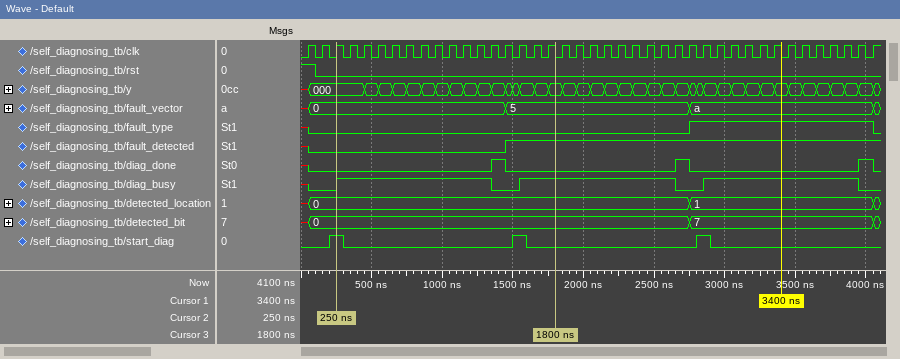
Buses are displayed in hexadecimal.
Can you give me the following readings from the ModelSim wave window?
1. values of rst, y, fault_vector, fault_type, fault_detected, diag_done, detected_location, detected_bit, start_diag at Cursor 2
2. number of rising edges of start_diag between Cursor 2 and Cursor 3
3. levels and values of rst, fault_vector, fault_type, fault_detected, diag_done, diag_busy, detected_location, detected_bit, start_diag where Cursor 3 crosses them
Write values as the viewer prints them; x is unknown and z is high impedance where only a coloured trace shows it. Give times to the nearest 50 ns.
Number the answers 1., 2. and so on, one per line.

1. rst=0, y=000, fault_vector=0, fault_type=0, fault_detected=0, diag_done=0, detected_location=0, detected_bit=0, start_diag=1
2. 1
3. rst=0, fault_vector=5, fault_type=0, fault_detected=1, diag_done=0, diag_busy=1, detected_location=0, detected_bit=0, start_diag=0
